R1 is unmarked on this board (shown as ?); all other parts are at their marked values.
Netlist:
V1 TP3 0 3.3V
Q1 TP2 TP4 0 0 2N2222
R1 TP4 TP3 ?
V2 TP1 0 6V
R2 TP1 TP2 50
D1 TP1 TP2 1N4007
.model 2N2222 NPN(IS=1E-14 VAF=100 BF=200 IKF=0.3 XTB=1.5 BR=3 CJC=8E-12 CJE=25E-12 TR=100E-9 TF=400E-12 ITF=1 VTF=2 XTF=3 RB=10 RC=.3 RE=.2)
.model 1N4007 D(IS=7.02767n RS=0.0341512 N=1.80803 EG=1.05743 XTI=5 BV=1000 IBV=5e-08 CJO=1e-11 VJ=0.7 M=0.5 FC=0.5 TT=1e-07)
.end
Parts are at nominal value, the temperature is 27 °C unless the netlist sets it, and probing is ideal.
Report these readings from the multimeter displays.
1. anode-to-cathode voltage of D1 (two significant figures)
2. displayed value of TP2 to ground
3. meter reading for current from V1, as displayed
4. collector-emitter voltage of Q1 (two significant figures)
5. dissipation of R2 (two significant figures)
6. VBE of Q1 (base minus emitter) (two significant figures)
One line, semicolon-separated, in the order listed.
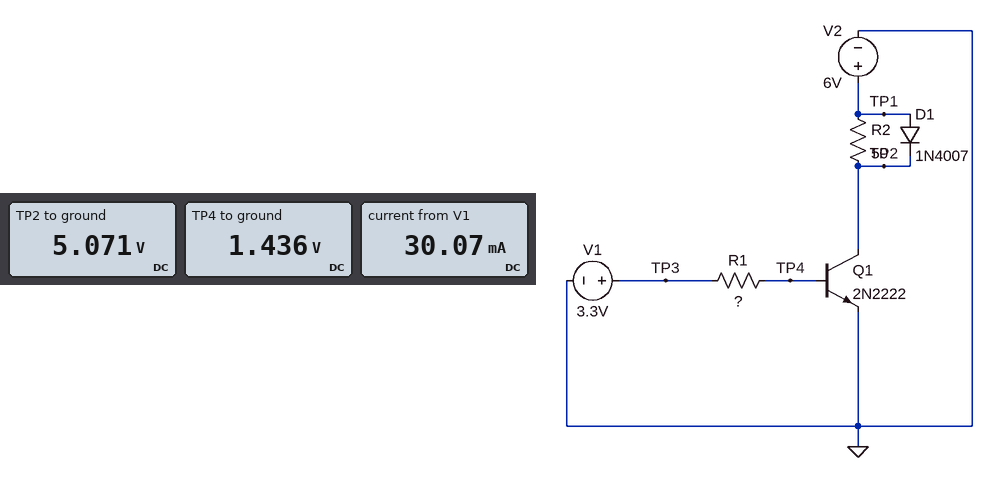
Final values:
930 mV; 5.071 V; 30.07 mA; 5.1 V; 17 mW; 1.4 V
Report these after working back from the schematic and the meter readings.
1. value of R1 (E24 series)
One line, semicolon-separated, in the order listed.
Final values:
62 Ω
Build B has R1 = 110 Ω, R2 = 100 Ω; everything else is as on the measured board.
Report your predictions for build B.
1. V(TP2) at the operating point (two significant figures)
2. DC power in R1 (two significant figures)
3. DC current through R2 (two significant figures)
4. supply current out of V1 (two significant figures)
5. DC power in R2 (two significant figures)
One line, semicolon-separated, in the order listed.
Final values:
5.1 V; 38 mW; 9.1 mA; 19 mA; 8.2 mW
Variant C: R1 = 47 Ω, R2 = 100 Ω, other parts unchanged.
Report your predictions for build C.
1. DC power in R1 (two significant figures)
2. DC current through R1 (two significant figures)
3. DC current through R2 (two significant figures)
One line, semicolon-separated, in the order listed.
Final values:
65 mW; 37 mA; 9.4 mA
